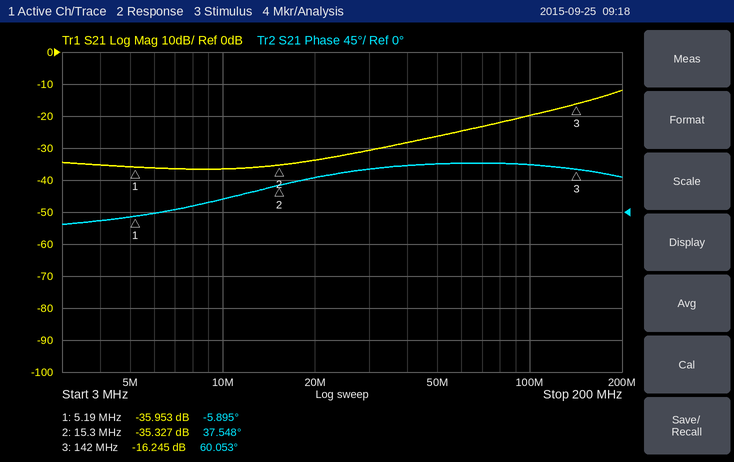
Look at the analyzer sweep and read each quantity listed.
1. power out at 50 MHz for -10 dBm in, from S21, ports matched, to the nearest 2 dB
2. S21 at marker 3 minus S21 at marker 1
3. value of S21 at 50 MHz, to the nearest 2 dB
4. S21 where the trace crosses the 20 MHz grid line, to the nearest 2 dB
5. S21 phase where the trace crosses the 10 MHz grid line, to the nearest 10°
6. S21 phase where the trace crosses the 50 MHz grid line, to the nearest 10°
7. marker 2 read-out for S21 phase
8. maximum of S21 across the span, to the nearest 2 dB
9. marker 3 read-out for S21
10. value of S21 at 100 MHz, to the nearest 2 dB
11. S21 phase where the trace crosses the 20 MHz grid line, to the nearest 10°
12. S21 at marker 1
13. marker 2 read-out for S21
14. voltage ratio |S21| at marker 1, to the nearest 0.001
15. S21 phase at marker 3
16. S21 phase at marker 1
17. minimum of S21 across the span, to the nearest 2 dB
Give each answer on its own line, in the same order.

-36 dBm
19.708 dB
-26 dB
-34 dB
20°
70°
37.548°
-12 dB
-16.245 dB
-20 dB
50°
-35.953 dB
-35.327 dB
0.016
60.053°
-5.895°
-36 dB
